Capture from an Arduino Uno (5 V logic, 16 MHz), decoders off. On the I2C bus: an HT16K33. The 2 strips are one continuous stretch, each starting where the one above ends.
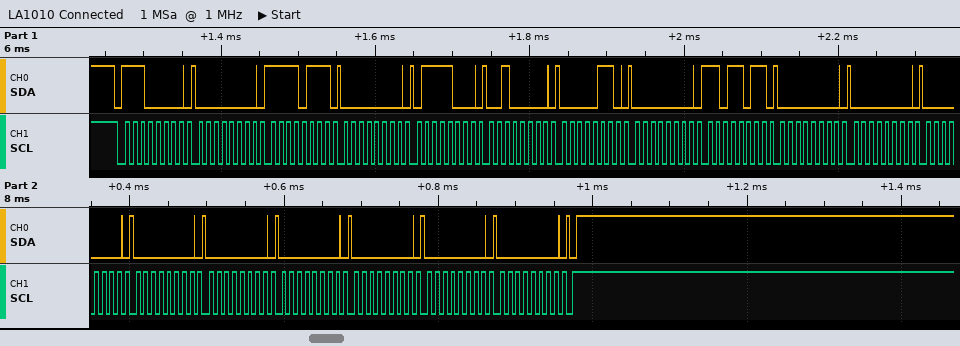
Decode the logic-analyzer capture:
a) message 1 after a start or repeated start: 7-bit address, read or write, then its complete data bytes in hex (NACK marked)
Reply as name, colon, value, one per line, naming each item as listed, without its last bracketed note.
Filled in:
message 1 after a start or repeated start: 7-bit address, read or write, then its complete data bytes in hex: 0x70 write: 00 F7 00 78 20 06 00 DB 00 00 00 00 00 00 00 00 00
